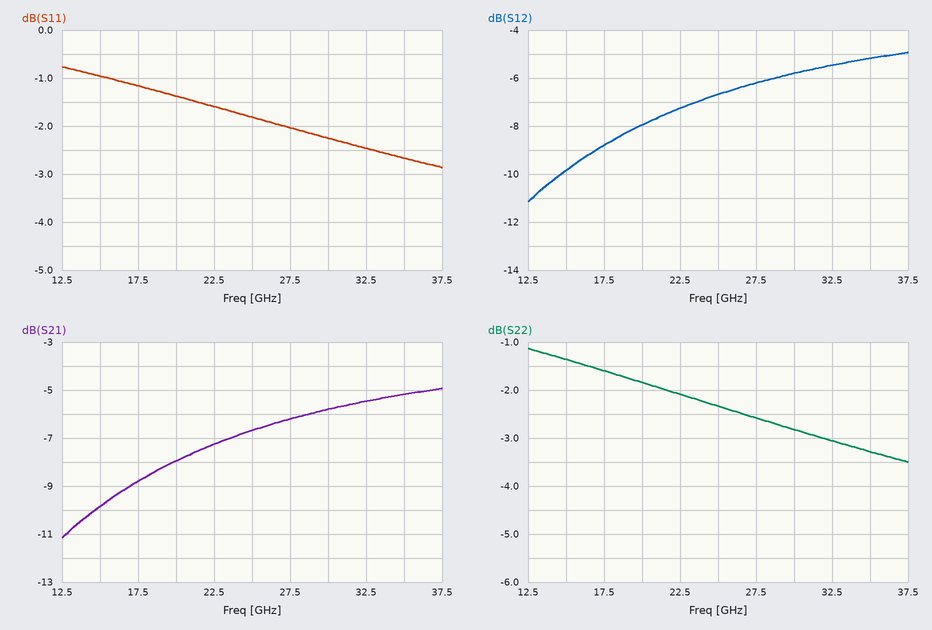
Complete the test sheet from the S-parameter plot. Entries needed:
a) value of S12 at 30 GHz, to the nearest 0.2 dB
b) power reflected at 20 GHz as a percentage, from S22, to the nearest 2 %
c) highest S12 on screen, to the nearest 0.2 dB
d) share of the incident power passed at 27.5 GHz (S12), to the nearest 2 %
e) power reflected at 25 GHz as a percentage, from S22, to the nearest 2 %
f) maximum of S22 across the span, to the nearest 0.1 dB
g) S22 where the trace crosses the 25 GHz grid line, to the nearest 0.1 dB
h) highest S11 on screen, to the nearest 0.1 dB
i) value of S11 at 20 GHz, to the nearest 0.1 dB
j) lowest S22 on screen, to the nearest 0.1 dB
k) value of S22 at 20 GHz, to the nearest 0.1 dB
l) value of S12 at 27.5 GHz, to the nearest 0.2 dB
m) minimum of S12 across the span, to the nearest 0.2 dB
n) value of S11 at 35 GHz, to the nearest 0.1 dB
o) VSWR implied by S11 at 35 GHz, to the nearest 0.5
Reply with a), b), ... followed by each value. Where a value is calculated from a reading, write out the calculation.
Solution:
a) -5.8 dB
b) 10^(-1.8/10) ≈ 66 %
c) -5.0 dB
d) 10^(-6.2/10) ≈ 24 %
e) 10^(-2.3/10) ≈ 58.9 %, so 58 % to the nearest 2 %
f) -1.1 dB
g) -2.3 dB
h) -0.8 dB
i) -1.4 dB
j) -3.5 dB
k) -1.8 dB
l) -6.2 dB
m) -11.2 dB
n) -2.7 dB
o) |Γ| = 10^(-2.7/20) = 0.7328; VSWR = (1 + 0.7328)/(1 − 0.7328) ≈ 6.5
